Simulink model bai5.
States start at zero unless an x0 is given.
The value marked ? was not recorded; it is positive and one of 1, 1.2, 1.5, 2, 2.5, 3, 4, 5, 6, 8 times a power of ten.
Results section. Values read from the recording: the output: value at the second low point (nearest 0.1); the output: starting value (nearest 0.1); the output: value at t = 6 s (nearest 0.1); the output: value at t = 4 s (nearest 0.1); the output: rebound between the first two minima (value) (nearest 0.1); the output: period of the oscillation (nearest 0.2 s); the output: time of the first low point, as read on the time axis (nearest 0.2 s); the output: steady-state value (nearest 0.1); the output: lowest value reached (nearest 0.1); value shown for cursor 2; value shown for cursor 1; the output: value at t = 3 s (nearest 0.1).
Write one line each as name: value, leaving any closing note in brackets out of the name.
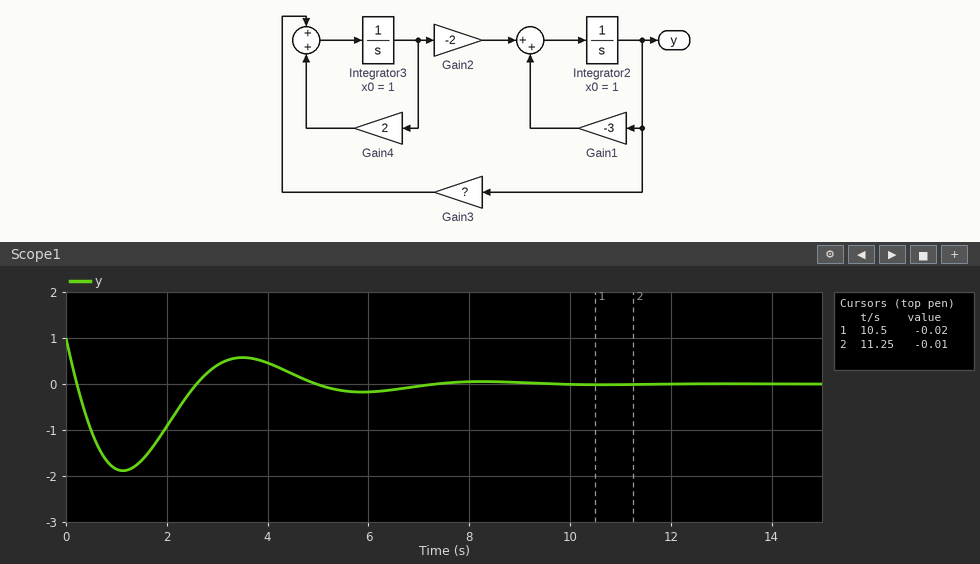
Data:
the output: value at the second low point: -0.2
the output: starting value: 1.0
the output: value at t = 6 s: -0.2
the output: value at t = 4 s: 0.5
the output: rebound between the first two minima (value): 0.6
the output: period of the oscillation: 4.8 s
the output: time of the first low point, as read on the time axis: 1.2 s
the output: steady-state value: 0.0
the output: lowest value reached: -1.9
value shown for cursor 2: -0.01
value shown for cursor 1: -0.02
the output: value at t = 3 s: 0.4
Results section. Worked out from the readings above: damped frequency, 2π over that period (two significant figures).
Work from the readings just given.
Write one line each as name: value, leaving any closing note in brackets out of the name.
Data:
damped frequency, 2π over that period: 1.3 rad/s
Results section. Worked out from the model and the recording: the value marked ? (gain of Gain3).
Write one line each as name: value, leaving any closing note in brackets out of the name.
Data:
the value marked ?: 4
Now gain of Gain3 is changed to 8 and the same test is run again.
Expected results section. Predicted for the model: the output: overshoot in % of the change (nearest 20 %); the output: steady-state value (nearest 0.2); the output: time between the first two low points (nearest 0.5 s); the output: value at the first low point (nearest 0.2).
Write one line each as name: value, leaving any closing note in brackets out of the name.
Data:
the output: overshoot in % of the change: 120 %
the output: steady-state value: 0.0
the output: time between the first two low points: 2.0 s
the output: value at the first low point: -1.2
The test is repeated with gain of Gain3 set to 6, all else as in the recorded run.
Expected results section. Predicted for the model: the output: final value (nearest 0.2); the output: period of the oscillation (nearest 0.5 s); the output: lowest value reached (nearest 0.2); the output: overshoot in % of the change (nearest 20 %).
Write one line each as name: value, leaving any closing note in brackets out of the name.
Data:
the output: final value: 0.0
the output: period of the oscillation: 2.5 s
the output: lowest value reached: -1.4
the output: overshoot in % of the change: 140 %
